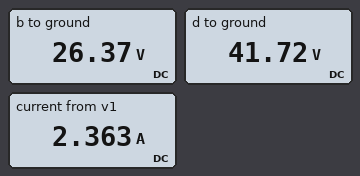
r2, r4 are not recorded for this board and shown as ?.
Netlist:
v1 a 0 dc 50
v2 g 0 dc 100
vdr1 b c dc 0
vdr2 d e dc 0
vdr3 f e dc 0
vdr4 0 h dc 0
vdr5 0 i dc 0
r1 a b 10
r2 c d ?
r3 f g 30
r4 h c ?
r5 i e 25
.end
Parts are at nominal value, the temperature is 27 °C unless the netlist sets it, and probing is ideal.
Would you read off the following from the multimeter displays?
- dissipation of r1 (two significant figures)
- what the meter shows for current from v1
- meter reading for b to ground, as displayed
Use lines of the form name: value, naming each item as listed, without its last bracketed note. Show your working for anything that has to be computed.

dissipation of r1: (50 V - 26.37 V)^2 / 10 Ω = 56 W
what the meter shows for current from v1: 2.363 A
meter reading for b to ground, as displayed: 26.37 V
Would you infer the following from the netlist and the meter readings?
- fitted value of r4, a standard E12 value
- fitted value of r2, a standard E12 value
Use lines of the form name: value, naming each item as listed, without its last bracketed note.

fitted value of r4, a standard E12 value: 10 Ω
fitted value of r2, a standard E12 value: 56 Ω
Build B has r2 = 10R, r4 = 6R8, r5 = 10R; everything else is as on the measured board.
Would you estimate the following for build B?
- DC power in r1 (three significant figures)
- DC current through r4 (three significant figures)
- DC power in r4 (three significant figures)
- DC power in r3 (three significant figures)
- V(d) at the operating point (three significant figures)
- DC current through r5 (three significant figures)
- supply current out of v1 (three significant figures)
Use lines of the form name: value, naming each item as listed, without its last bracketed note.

DC power in r1: 83.3 W
DC current through r4: 3.11 A
DC power in r4: 65.7 W
DC power in r3: 196 W
V(d) at the operating point: 23.3 V
DC current through r5: 2.33 A
supply current out of v1: 2.89 A
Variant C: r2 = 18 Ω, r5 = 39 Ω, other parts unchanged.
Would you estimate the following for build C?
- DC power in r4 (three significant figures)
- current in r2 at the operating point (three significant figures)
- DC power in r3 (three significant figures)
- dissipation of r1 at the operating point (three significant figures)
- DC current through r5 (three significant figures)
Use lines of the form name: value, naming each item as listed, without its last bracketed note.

DC power in r4: 83.8 W
current in r2 at the operating point: 789 mA
DC power in r3: 108 W
dissipation of r1 at the operating point: 44.3 W
DC current through r5: 1.11 A
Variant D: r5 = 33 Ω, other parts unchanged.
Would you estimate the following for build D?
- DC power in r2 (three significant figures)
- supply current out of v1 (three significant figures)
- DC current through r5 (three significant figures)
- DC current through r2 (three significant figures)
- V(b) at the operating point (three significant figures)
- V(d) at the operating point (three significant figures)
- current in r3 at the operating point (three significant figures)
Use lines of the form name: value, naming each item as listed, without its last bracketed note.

DC power in r2: 7.13 W
supply current out of v1: 2.32 A
DC current through r5: 1.42 A
DC current through r2: 357 mA
V(b) at the operating point: 26.8 V
V(d) at the operating point: 46.8 V
current in r3 at the operating point: 1.77 A
